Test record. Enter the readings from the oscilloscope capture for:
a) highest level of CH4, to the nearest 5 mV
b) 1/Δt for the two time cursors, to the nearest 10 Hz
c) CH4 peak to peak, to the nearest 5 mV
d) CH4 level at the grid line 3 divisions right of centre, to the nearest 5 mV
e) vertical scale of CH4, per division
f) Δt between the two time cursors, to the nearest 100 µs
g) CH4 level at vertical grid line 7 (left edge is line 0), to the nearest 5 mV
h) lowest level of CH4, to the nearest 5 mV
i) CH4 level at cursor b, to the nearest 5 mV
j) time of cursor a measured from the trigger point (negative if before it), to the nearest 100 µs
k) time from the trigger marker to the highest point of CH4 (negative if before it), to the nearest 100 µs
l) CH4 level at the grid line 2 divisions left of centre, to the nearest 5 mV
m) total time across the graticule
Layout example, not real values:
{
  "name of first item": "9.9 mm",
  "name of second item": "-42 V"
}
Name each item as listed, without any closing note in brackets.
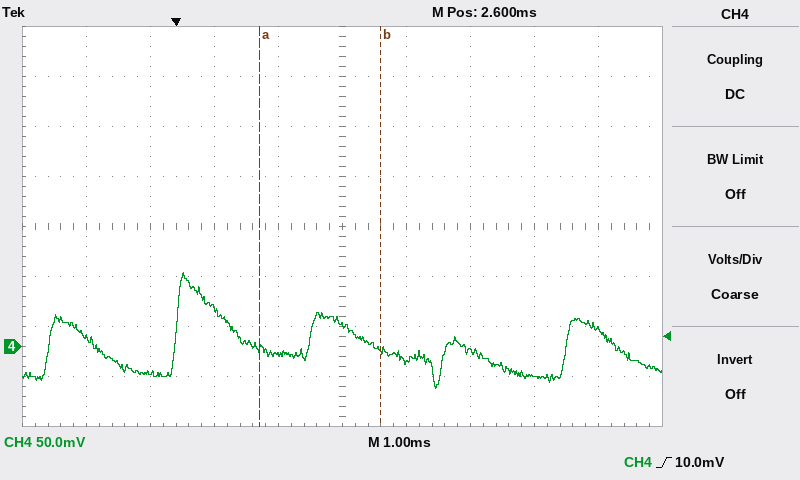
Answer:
{
  "highest level of CH4, to the nearest 5 mV": "75 mV",
  "1/Δt for the two time cursors, to the nearest 10 Hz": "530 Hz",
  "CH4 peak to peak, to the nearest 5 mV": "115 mV",
  "CH4 level at the grid line 3 divisions right of centre, to the nearest 5 mV": "-30 mV",
  "vertical scale of CH4, per division": "50 mV",
  "Δt between the two time cursors, to the nearest 100 µs": "1.9 ms",
  "CH4 level at vertical grid line 7 (left edge is line 0), to the nearest 5 mV": "-5 mV",
  "lowest level of CH4, to the nearest 5 mV": "-40 mV",
  "CH4 level at cursor b, to the nearest 5 mV": "-5 mV",
  "time of cursor a measured from the trigger point (negative if before it), to the nearest 100 µs": "+1.3 ms",
  "time from the trigger marker to the highest point of CH4 (negative if before it), to the nearest 100 µs": "+100 µs",
  "CH4 level at the grid line 2 divisions left of centre, to the nearest 5 mV": "40 mV",
  "total time across the graticule": "10 ms"
}
